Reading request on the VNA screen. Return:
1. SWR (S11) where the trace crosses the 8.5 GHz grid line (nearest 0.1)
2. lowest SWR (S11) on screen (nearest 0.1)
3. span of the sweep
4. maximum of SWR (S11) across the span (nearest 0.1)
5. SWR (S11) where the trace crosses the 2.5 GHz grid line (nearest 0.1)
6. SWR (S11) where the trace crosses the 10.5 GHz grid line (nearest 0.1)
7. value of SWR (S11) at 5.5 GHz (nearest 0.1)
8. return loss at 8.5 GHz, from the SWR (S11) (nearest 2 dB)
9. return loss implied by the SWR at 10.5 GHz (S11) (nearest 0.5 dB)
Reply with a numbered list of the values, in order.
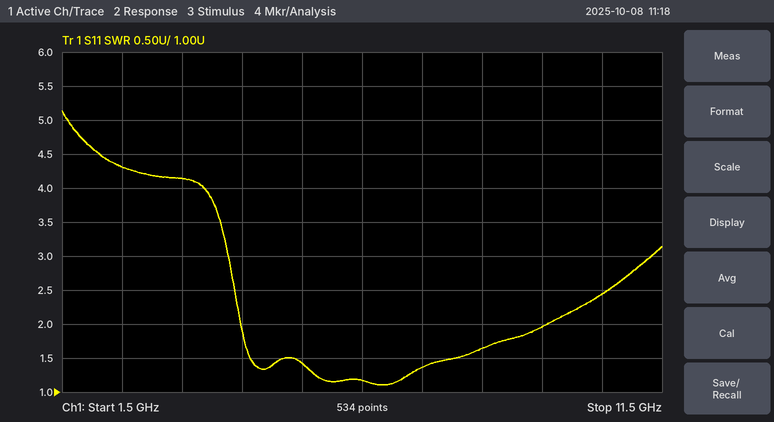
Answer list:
1. 1.6
2. 1.1
3. 10 GHz
4. 5.1
5. 4.3
6. 2.4
7. 1.4
8. 12 dB
9. 7.5 dB
